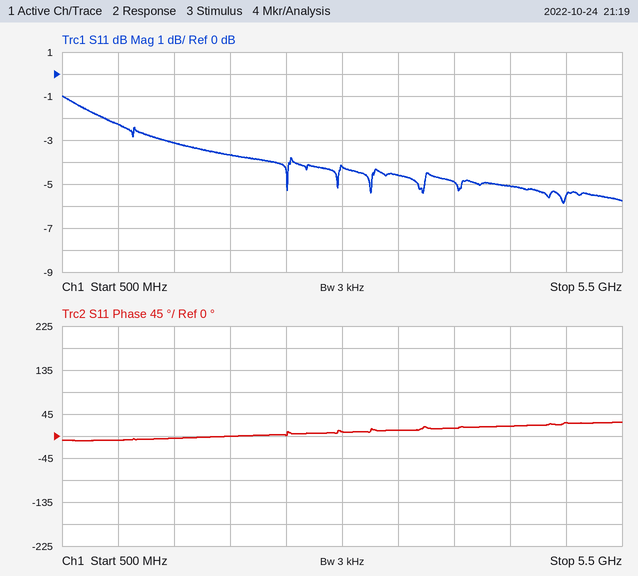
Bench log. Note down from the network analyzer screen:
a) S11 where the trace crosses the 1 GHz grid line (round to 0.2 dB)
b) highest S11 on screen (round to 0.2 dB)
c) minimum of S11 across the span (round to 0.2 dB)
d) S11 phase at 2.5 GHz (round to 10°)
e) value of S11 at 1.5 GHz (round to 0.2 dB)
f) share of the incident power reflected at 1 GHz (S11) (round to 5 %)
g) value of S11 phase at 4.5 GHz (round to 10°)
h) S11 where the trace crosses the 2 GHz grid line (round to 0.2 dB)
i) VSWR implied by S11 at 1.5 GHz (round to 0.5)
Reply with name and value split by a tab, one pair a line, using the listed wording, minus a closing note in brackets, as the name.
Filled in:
S11 where the trace crosses the 1 GHz grid line	-2.2 dB
highest S11 on screen	-1.0 dB
minimum of S11 across the span	-5.8 dB
S11 phase at 2.5 GHz	0°
value of S11 at 1.5 GHz	-3.2 dB
share of the incident power reflected at 1 GHz (S11)	60 %
value of S11 phase at 4.5 GHz	20°
S11 where the trace crosses the 2 GHz grid line	-3.6 dB
VSWR implied by S11 at 1.5 GHz	5.5
